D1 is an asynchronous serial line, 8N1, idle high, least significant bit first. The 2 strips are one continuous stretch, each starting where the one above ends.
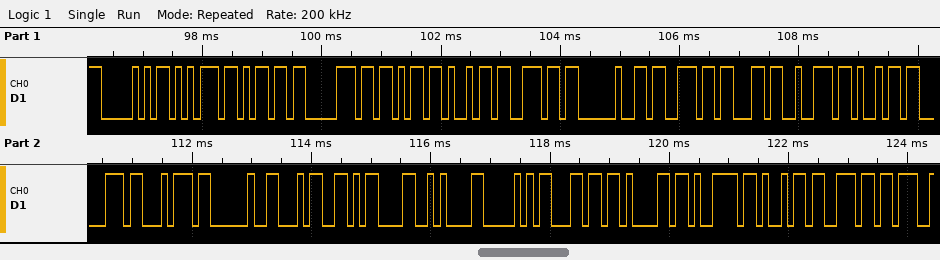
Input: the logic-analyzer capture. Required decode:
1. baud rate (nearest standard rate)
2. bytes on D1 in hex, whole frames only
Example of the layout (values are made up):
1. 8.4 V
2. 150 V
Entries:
1. 9600 baud
2. 50 75 6D 70 6B 69 6E 20 73 63 72 69 70 74 20 34 0D 0A 50 6C 61 79 69 6E
